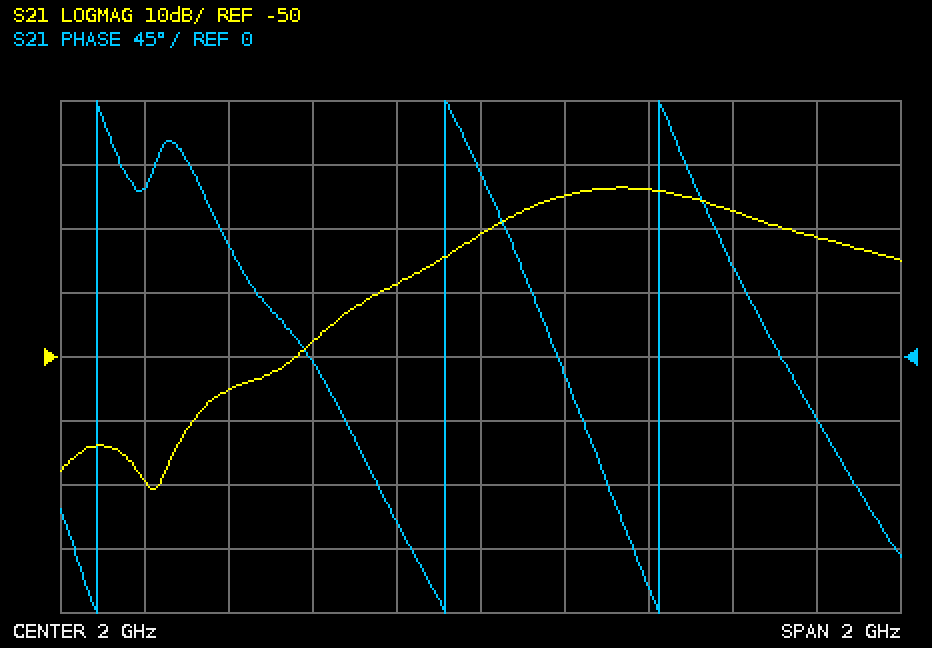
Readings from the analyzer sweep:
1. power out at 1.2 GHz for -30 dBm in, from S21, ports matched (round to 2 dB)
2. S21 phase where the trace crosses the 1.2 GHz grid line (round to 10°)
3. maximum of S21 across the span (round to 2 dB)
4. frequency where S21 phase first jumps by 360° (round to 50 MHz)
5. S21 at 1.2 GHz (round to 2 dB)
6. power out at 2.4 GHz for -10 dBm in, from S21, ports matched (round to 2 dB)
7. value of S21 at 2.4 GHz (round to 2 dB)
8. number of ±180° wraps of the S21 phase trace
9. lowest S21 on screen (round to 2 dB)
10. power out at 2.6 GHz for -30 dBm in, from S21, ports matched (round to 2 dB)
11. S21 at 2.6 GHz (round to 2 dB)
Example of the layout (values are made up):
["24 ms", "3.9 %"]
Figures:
["-100 dBm", "120°", "-24 dB", "1.10 GHz", "-70 dB", "-34 dBm", "-24 dB", "3", "-70 dB", "-58 dBm", "-28 dB"]
